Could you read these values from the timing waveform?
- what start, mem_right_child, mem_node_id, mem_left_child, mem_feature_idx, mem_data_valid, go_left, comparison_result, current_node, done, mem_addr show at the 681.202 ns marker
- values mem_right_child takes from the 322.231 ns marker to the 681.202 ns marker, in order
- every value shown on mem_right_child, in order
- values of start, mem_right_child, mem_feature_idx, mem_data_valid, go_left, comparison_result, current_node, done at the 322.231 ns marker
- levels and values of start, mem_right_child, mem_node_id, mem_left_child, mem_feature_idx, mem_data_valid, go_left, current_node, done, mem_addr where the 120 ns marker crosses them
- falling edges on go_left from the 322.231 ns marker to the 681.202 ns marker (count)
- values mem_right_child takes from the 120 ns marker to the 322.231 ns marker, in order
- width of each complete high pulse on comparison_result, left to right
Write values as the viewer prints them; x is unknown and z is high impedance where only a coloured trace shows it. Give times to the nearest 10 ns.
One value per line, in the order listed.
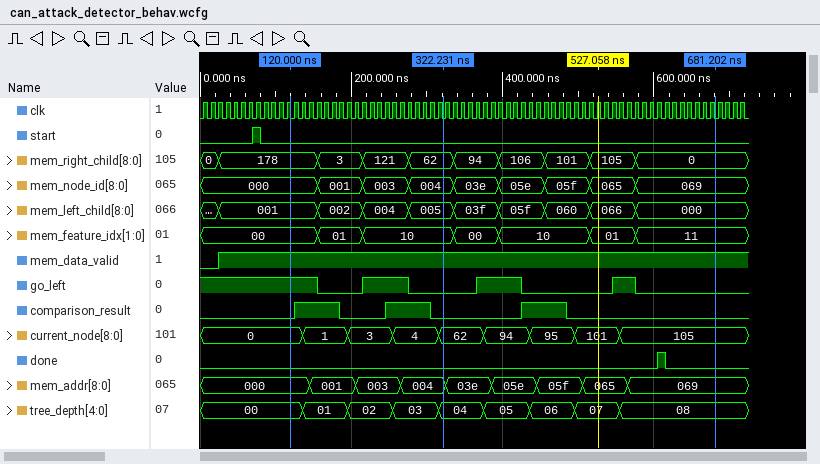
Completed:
start=0, mem_right_child=0, mem_node_id=069, mem_left_child=000, mem_feature_idx=11, mem_data_valid=1, go_left=0, comparison_result=0, current_node=105, done=0, mem_addr=069
62, 94, 106, 101, 105, 0
0, 178, 3, 121, 62, 94, 106, 101, 105, 0
start=0, mem_right_child=62, mem_feature_idx=10, mem_data_valid=1, go_left=0, comparison_result=0, current_node=62, done=0
start=0, mem_right_child=178, mem_node_id=000, mem_left_child=001, mem_feature_idx=00, mem_data_valid=1, go_left=1, current_node=0, done=0, mem_addr=000
2
178, 3, 121, 62
60 ns, 60 ns, 60 ns
